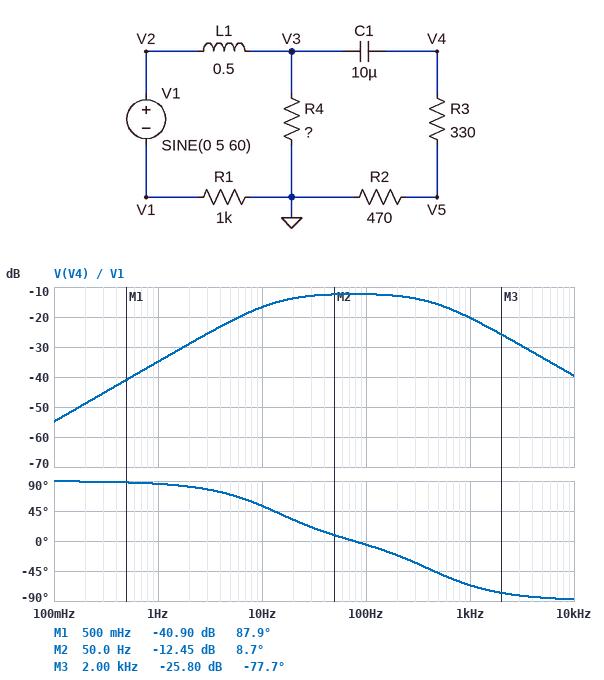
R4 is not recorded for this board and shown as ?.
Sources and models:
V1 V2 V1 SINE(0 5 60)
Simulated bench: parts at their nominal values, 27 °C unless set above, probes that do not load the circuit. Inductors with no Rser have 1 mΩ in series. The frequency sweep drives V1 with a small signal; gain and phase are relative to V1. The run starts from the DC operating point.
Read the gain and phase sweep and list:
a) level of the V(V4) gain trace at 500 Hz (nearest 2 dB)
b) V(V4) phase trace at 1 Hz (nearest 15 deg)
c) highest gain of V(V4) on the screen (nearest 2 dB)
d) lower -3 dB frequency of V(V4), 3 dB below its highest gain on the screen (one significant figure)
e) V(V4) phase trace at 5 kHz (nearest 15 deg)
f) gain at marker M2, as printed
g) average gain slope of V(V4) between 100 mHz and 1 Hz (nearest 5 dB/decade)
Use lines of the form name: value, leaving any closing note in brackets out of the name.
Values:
level of the V(V4) gain trace at 500 Hz: -16 dB
V(V4) phase trace at 1 Hz: 90 deg
highest gain of V(V4) on the screen: -12 dB
lower -3 dB frequency of V(V4), 3 dB below its highest gain on the screen: 10 Hz
V(V4) phase trace at 5 kHz: -90 deg
gain at marker M2, as printed: -12.45 dB
average gain slope of V(V4) between 100 mHz and 1 Hz: 20 dB/decade
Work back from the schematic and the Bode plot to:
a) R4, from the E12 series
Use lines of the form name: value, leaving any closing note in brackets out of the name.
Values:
R4, from the E12 series: 560 Ω
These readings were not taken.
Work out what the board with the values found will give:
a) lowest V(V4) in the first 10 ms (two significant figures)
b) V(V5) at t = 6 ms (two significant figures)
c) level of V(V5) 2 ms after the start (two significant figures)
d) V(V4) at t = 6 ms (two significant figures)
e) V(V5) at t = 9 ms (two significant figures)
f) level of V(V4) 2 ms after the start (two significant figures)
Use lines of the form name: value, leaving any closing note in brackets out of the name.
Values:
lowest V(V4) in the first 10 ms: -900 mV
V(V5) at t = 6 ms: 410 mV
level of V(V5) 2 ms after the start: 390 mV
V(V4) at t = 6 ms: 690 mV
V(V5) at t = 9 ms: -310 mV
level of V(V4) 2 ms after the start: 660 mV
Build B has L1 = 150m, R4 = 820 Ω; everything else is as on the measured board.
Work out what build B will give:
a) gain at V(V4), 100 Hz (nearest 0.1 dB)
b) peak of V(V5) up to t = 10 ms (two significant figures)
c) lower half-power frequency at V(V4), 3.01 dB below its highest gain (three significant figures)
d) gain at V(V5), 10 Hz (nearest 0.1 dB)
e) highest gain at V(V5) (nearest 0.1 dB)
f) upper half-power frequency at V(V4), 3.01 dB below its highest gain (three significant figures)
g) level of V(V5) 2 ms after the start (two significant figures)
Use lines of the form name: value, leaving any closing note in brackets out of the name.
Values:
gain at V(V4), 100 Hz: -10.9 dB
peak of V(V5) up to t = 10 ms: 700 mV
lower half-power frequency at V(V4), 3.01 dB below its highest gain: 12.5 Hz
gain at V(V5), 10 Hz: -19.6 dB
highest gain at V(V5): -15.5 dB
upper half-power frequency at V(V4), 3.01 dB below its highest gain: 1.51 kHz
level of V(V5) 2 ms after the start: 510 mV
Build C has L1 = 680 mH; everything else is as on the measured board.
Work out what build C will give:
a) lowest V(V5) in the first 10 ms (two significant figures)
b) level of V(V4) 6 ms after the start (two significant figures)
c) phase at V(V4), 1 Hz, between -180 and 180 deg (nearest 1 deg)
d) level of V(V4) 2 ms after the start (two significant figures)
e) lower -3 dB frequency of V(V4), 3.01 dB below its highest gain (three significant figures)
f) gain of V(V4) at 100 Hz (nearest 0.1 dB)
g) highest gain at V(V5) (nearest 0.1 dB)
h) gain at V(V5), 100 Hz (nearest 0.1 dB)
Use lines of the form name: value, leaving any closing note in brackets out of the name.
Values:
lowest V(V5) in the first 10 ms: -500 mV
level of V(V4) 6 ms after the start: 720 mV
phase at V(V4), 1 Hz, between -180 and 180 deg: 86 deg
level of V(V4) 2 ms after the start: 610 mV
lower -3 dB frequency of V(V4), 3.01 dB below its highest gain: 12.7 Hz
gain of V(V4) at 100 Hz: -12.6 dB
highest gain at V(V5): -17.1 dB
gain at V(V5), 100 Hz: -17.2 dB
